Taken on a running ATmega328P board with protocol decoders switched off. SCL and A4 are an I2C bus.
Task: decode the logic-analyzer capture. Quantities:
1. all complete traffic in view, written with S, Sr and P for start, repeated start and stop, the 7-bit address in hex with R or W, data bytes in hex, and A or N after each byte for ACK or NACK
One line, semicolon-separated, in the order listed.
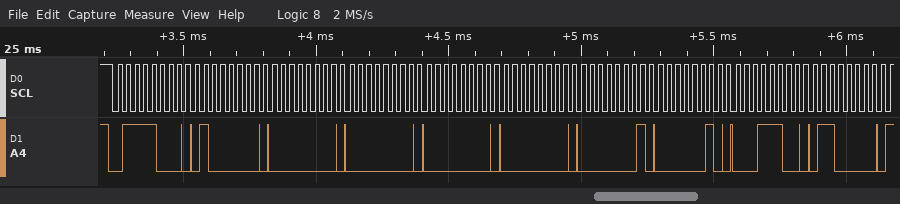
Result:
S 3CW A 40 A 00 A 00 A 00 A 00 A 01 A 02 A 1C A 60 A
